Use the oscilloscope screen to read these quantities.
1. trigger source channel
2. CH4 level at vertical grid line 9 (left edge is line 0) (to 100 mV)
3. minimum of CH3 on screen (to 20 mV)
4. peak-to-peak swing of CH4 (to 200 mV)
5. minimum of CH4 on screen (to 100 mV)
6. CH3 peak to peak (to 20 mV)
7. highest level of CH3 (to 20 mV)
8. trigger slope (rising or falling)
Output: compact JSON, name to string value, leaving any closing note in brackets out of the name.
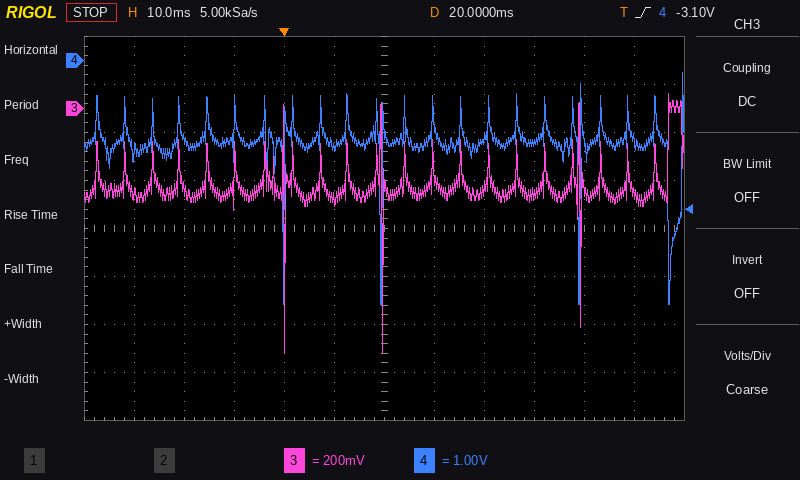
{"trigger source channel": "CH4", "CH4 level at vertical grid line 9 (left edge is line 0)": "-1.7 V", "minimum of CH3 on screen": "-1.02 V", "peak-to-peak swing of CH4": "4.8 V", "minimum of CH4 on screen": "-5.1 V", "CH3 peak to peak": "1.08 V", "highest level of CH3": "60 mV", "trigger slope": "rising"}
